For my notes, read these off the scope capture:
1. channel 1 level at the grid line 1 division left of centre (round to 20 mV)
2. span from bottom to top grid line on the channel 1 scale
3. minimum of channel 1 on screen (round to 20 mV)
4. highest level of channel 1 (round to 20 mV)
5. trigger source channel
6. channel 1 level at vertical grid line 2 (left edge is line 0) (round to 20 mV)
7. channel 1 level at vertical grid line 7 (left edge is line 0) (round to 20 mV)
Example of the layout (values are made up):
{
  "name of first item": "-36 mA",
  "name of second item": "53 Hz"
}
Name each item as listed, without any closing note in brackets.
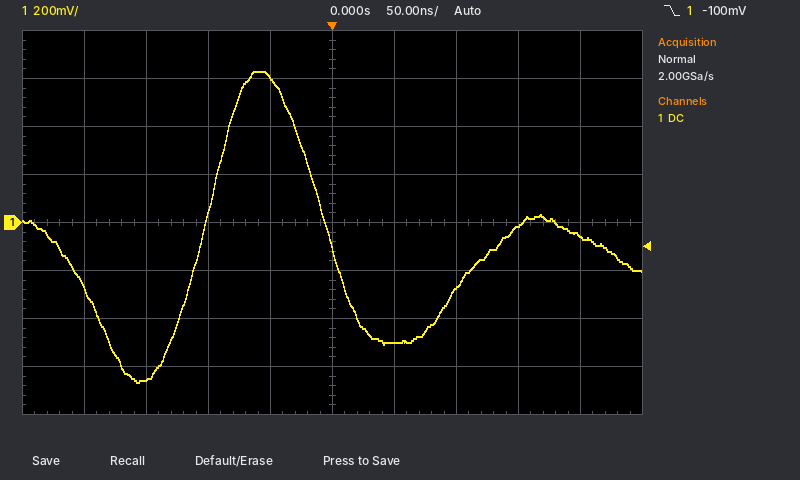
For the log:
{
  "channel 1 level at the grid line 1 division left of centre": "600 mV",
  "span from bottom to top grid line on the channel 1 scale": "1.6 V",
  "minimum of channel 1 on screen": "-660 mV",
  "highest level of channel 1": "620 mV",
  "trigger source channel": "channel 1",
  "channel 1 level at vertical grid line 2 (left edge is line 0)": "-660 mV",
  "channel 1 level at vertical grid line 7 (left edge is line 0)": "-280 mV"
}
